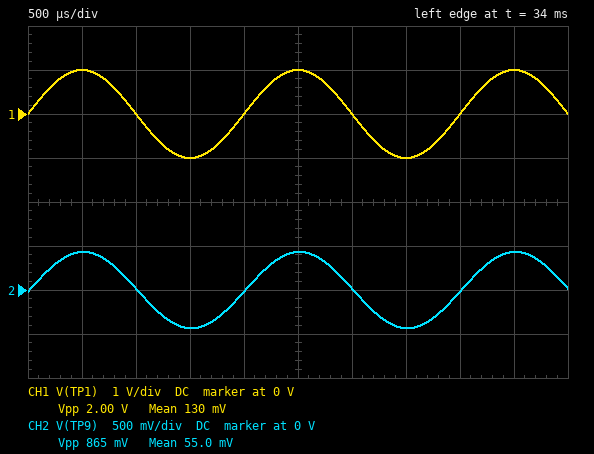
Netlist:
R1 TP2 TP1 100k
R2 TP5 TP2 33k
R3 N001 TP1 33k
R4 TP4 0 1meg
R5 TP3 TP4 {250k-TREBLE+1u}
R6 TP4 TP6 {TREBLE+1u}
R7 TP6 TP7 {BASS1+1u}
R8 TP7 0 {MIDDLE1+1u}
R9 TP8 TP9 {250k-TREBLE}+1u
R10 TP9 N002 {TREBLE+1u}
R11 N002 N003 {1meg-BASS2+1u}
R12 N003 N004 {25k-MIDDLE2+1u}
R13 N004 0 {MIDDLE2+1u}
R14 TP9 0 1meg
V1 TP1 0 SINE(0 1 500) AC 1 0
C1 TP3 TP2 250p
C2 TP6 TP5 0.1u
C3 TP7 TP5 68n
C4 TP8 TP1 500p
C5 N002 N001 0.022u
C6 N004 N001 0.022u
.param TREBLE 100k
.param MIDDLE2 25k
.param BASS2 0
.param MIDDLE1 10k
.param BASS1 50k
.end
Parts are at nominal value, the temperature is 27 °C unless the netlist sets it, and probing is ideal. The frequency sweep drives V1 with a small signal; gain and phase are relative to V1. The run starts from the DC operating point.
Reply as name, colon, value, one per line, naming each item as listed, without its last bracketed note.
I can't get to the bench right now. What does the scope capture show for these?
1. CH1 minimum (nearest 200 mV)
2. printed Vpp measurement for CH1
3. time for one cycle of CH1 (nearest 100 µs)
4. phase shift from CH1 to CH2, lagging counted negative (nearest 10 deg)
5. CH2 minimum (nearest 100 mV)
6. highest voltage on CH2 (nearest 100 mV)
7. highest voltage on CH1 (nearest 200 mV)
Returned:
CH1 minimum: -1.0 V
printed Vpp measurement for CH1: 2.00 V
time for one cycle of CH1: 2.0 ms
phase shift from CH1 to CH2, lagging counted negative: 0 deg
CH2 minimum: -400 mV
highest voltage on CH2: 400 mV
highest voltage on CH1: 1.0 V
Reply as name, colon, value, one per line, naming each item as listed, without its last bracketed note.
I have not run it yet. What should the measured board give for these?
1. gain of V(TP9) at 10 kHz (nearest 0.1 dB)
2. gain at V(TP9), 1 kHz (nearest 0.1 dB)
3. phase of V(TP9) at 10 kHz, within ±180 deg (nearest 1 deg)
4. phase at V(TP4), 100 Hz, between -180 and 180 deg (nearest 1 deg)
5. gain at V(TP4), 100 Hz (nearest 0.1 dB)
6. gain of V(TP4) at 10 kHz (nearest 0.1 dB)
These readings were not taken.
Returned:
gain of V(TP9) at 10 kHz: -0.4 dB
gain at V(TP9), 1 kHz: -6.7 dB
phase of V(TP9) at 10 kHz, within ±180 deg: 10 deg
phase at V(TP4), 100 Hz, between -180 and 180 deg: -25 deg
gain at V(TP4), 100 Hz: -16.4 dB
gain of V(TP4) at 10 kHz: -17.0 dB
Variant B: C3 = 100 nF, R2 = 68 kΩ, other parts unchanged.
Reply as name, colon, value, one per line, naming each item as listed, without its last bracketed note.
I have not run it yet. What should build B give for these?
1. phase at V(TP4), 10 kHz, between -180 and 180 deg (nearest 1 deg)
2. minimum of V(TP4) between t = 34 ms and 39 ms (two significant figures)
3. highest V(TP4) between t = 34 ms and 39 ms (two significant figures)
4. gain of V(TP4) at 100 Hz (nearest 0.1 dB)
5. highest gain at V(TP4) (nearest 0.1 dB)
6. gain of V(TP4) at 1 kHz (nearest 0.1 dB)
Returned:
phase at V(TP4), 10 kHz, between -180 and 180 deg: 9 deg
minimum of V(TP4) between t = 34 ms and 39 ms: -61 mV
highest V(TP4) between t = 34 ms and 39 ms: 60 mV
gain of V(TP4) at 100 Hz: -20.1 dB
highest gain at V(TP4): -14.9 dB
gain of V(TP4) at 1 kHz: -21.6 dB
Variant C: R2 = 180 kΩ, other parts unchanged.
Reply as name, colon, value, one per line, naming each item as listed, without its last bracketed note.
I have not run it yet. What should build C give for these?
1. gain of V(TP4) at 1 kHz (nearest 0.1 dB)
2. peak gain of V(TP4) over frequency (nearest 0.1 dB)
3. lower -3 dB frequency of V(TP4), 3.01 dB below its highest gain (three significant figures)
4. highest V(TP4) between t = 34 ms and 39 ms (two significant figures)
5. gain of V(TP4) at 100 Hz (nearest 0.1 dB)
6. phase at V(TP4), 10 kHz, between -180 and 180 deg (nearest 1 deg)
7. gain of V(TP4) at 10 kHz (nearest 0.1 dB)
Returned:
gain of V(TP4) at 1 kHz: -20.2 dB
peak gain of V(TP4) over frequency: -13.0 dB
lower -3 dB frequency of V(TP4), 3.01 dB below its highest gain: 2.08 kHz
highest V(TP4) between t = 34 ms and 39 ms: 55 mV
gain of V(TP4) at 100 Hz: -22.6 dB
phase at V(TP4), 10 kHz, between -180 and 180 deg: 10 deg
gain of V(TP4) at 10 kHz: -13.1 dB
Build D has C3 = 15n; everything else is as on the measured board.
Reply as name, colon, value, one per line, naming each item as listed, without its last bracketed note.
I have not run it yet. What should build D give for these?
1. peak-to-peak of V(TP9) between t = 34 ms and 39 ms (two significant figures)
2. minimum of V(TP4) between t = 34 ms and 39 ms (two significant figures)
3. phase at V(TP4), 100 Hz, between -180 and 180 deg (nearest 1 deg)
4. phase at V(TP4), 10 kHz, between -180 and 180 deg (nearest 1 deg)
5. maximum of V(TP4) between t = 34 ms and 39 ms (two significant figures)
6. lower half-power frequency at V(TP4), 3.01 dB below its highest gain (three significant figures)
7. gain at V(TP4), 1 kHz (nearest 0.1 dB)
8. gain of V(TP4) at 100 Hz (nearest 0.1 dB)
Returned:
peak-to-peak of V(TP9) between t = 34 ms and 39 ms: 870 mV
minimum of V(TP4) between t = 34 ms and 39 ms: -140 mV
phase at V(TP4), 100 Hz, between -180 and 180 deg: -8 deg
phase at V(TP4), 10 kHz, between -180 and 180 deg: 5 deg
maximum of V(TP4) between t = 34 ms and 39 ms: 140 mV
lower half-power frequency at V(TP4), 3.01 dB below its highest gain: 7.36 Hz
gain at V(TP4), 1 kHz: -20.3 dB
gain of V(TP4) at 100 Hz: -12.2 dB
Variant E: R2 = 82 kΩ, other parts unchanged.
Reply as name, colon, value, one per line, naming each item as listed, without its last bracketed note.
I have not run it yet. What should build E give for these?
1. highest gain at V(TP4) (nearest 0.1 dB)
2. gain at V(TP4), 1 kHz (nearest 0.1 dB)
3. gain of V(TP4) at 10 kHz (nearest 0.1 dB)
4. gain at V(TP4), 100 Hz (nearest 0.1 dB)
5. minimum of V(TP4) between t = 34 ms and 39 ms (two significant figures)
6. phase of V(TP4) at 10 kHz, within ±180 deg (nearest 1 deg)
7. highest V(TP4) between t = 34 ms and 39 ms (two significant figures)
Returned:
highest gain at V(TP4): -14.5 dB
gain at V(TP4), 1 kHz: -21.5 dB
gain of V(TP4) at 10 kHz: -14.7 dB
gain at V(TP4), 100 Hz: -19.0 dB
minimum of V(TP4) between t = 34 ms and 39 ms: -60 mV
phase of V(TP4) at 10 kHz, within ±180 deg: 9 deg
highest V(TP4) between t = 34 ms and 39 ms: 59 mV
